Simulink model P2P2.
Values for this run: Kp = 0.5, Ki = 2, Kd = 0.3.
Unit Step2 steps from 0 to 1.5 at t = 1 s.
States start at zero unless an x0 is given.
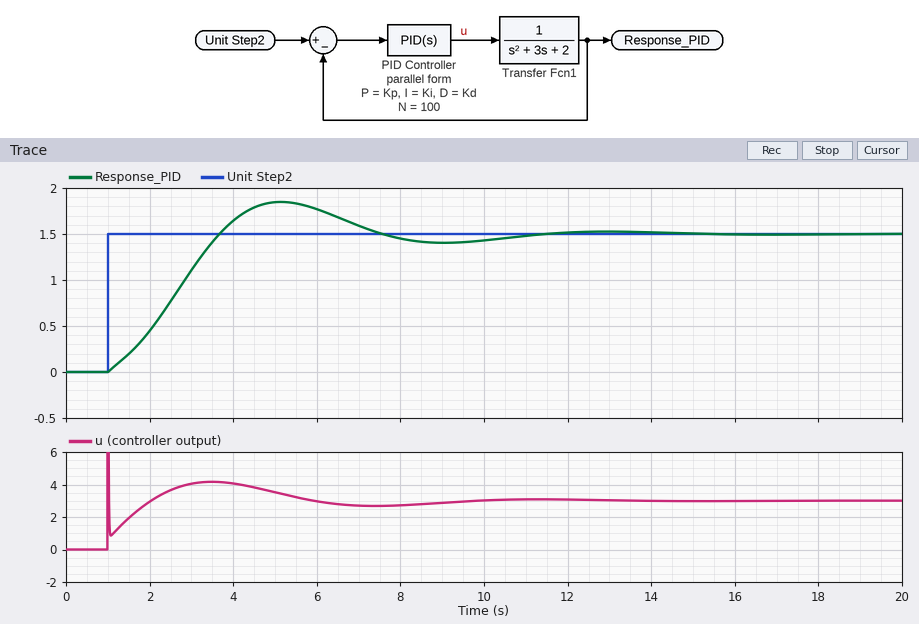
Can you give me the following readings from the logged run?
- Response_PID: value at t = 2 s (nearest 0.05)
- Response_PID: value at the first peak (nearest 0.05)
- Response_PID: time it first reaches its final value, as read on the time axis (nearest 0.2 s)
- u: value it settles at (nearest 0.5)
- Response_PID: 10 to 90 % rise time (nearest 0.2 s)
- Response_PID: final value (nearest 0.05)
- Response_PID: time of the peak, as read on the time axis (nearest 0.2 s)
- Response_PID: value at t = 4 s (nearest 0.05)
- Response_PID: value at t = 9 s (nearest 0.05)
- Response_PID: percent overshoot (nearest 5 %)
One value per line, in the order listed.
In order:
0.45
1.85
3.6 s
3.0
2.0 s
1.50
5.2 s
1.65
1.40
25 %
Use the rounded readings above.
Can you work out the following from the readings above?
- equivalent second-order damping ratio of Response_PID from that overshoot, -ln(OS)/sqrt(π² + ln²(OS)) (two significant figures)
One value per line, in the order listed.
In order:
0.40
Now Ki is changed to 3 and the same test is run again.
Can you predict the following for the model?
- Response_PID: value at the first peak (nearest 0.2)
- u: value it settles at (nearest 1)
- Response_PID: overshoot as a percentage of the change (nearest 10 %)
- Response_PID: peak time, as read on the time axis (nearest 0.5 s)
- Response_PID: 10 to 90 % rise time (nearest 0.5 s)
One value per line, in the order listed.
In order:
2.0
3
40 %
4.5 s
1.5 s
